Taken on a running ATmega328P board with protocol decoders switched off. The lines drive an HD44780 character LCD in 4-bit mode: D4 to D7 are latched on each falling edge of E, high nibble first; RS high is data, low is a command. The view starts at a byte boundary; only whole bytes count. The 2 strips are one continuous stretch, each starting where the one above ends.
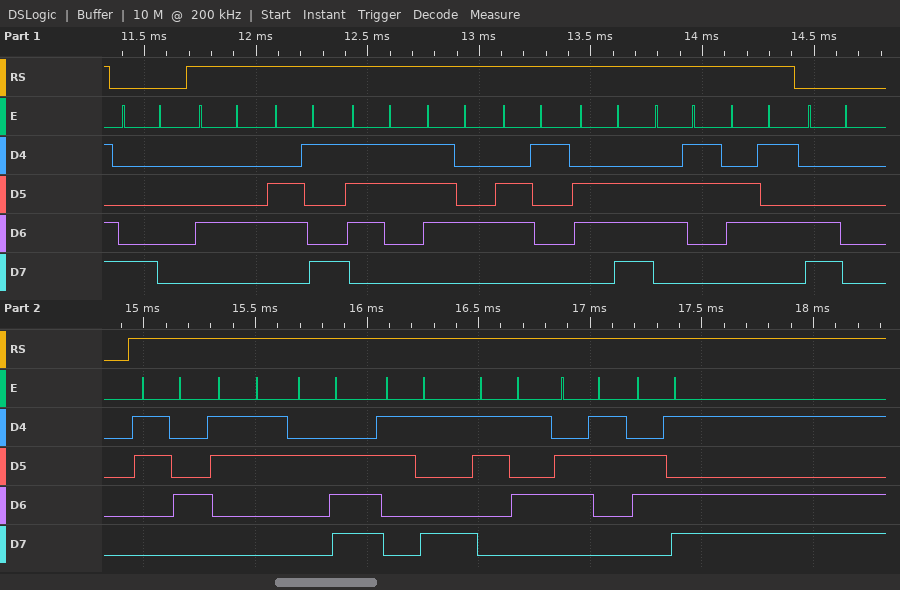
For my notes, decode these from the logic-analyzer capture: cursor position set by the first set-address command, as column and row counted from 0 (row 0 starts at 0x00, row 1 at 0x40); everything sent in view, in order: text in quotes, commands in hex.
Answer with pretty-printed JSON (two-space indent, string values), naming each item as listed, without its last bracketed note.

{
  "cursor position set by the first set-address command, as column and row counted from 0": "column 0, row 0",
  "everything sent in view, in order: text in quotes, commands in hex": "0x80 \"Distance\" 0xC0 \"43.95cm\""
}
